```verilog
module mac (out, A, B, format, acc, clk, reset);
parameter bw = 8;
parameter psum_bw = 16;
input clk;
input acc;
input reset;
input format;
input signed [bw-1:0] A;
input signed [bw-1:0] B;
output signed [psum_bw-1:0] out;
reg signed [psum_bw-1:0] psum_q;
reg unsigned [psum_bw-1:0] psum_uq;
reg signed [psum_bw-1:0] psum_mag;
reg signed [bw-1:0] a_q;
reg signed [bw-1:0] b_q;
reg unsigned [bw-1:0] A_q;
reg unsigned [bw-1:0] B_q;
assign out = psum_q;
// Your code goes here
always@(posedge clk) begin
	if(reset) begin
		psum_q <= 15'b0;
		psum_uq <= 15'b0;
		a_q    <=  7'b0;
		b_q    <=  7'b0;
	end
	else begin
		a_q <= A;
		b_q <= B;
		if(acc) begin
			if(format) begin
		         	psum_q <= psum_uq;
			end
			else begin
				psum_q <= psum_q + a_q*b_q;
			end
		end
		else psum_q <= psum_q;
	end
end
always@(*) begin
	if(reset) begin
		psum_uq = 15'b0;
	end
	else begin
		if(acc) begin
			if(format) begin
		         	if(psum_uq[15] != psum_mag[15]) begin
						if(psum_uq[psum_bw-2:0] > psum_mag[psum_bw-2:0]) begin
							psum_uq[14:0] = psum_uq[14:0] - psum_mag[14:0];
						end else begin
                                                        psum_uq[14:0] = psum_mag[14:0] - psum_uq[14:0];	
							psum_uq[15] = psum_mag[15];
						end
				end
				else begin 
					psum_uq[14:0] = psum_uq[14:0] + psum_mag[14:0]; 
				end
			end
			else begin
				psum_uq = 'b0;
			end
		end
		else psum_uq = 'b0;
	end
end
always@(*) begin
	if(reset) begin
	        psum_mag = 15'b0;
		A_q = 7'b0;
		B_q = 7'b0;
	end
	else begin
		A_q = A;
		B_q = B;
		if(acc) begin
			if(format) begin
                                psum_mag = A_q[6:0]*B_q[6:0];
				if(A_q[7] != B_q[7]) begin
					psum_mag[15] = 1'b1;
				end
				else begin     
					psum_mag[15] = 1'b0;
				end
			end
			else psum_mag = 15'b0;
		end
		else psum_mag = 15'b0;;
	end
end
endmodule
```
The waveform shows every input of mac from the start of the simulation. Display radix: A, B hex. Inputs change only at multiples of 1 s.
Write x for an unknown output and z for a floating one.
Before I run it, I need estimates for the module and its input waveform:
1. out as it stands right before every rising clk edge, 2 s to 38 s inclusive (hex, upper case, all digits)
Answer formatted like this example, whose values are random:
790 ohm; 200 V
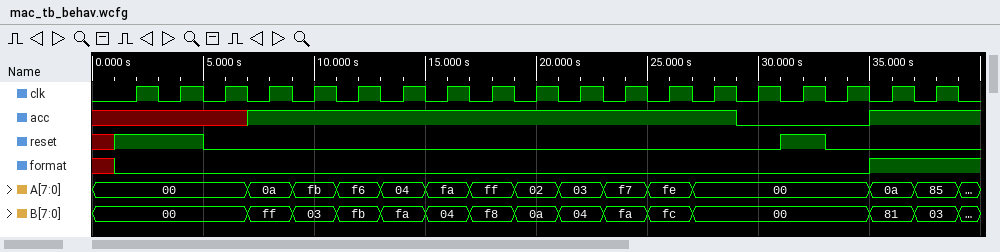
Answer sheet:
x, 0000, 0000, 0000, 0000, FFF6, FFE7, 0019, 0001, FFE9, FFF1, 0005, 0011, 0047, 004F, 004F, 0000, 0000, 800A
